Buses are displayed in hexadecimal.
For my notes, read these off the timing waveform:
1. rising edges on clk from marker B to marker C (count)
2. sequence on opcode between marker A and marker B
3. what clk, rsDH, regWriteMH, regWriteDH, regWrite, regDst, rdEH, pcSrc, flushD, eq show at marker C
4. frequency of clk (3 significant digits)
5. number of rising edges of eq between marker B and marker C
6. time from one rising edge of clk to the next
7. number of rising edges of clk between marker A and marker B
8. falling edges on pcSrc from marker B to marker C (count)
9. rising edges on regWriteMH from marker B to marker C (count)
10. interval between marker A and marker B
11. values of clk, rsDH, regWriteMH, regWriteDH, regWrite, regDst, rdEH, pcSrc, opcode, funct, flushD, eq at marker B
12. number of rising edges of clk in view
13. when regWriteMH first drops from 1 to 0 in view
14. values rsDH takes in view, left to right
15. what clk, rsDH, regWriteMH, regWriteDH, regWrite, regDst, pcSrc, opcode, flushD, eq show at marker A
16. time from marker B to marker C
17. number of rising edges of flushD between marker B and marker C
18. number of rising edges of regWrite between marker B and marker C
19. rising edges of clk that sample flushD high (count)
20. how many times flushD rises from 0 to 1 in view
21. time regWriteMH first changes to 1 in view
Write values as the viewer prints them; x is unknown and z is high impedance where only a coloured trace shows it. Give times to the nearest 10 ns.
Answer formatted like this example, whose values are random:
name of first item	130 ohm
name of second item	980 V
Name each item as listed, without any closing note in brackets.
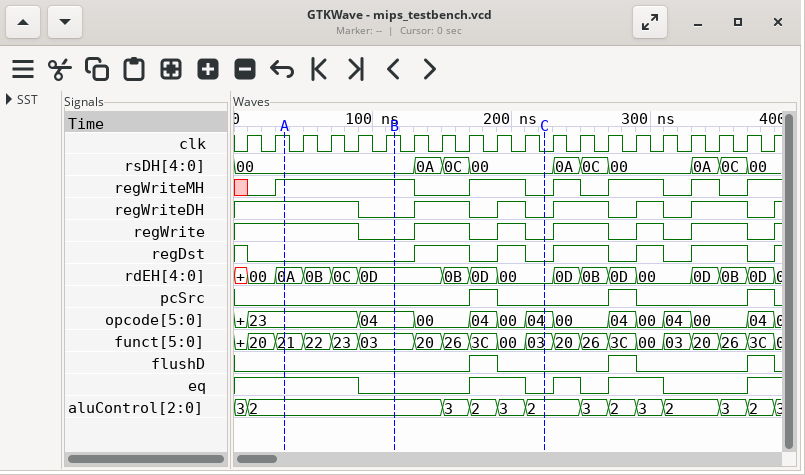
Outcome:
rising edges on clk from marker B to marker C	5
sequence on opcode between marker A and marker B	23, 04
what clk, rsDH, regWriteMH, regWriteDH, regWrite, regDst, rdEH, pcSrc, flushD, eq show at marker C	clk=0, rsDH=00, regWriteMH=0, regWriteDH=0, regWrite=0, regDst=0, rdEH=00, pcSrc=0, flushD=0, eq=0
frequency of clk	50.0 MHz
number of rising edges of eq between marker B and marker C	1
time from one rising edge of clk to the next	20 ns
number of rising edges of clk between marker A and marker B	4
falling edges on pcSrc from marker B to marker C	1
rising edges on regWriteMH from marker B to marker C	1
interval between marker A and marker B	80 ns
values of clk, rsDH, regWriteMH, regWriteDH, regWrite, regDst, rdEH, pcSrc, opcode, funct, flushD, eq at marker B	clk=1, rsDH=00, regWriteMH=1, regWriteDH=0, regWrite=0, regDst=0, rdEH=0D, pcSrc=0, opcode=04, funct=03, flushD=0, eq=0
number of rising edges of clk in view	20
when regWriteMH first drops from 1 to 0 in view	130 ns
values rsDH takes in view, left to right	00, 0A, 0C, 00, 0A, 0C, 00, 0A, 0C, 00
what clk, rsDH, regWriteMH, regWriteDH, regWrite, regDst, pcSrc, opcode, flushD, eq show at marker A	clk=1, rsDH=00, regWriteMH=1, regWriteDH=1, regWrite=1, regDst=0, pcSrc=0, opcode=23, flushD=0, eq=1
time from marker B to marker C	110 ns
number of rising edges of flushD between marker B and marker C	1
number of rising edges of regWrite between marker B and marker C	2
rising edges of clk that sample flushD high	3
how many times flushD rises from 0 to 1 in view	3
time regWriteMH first changes to 1 in view	30 ns
